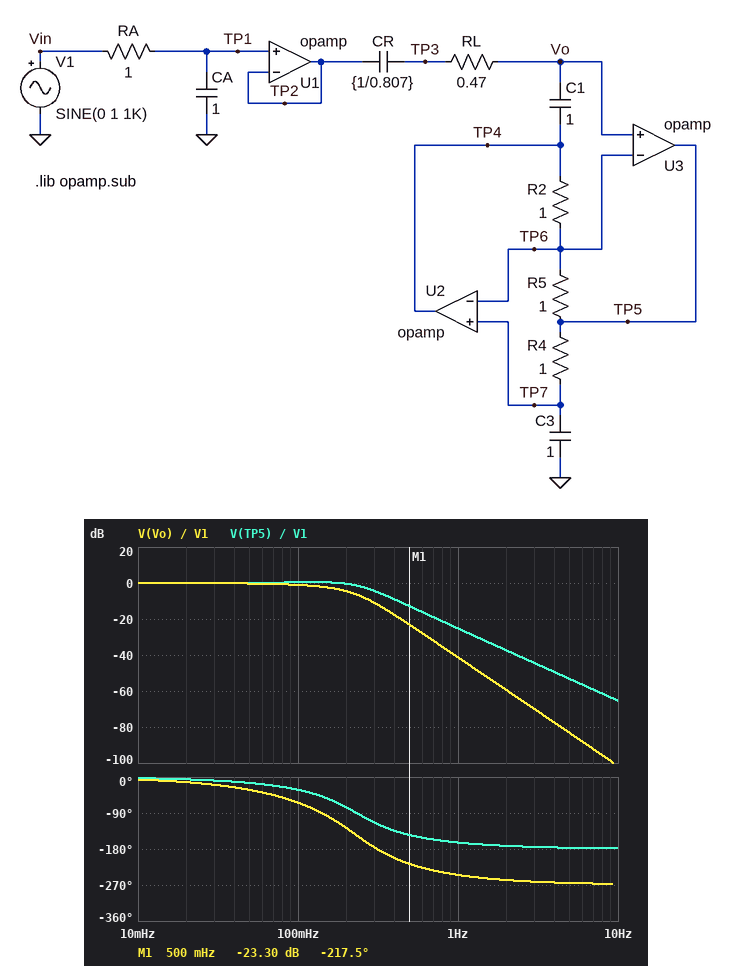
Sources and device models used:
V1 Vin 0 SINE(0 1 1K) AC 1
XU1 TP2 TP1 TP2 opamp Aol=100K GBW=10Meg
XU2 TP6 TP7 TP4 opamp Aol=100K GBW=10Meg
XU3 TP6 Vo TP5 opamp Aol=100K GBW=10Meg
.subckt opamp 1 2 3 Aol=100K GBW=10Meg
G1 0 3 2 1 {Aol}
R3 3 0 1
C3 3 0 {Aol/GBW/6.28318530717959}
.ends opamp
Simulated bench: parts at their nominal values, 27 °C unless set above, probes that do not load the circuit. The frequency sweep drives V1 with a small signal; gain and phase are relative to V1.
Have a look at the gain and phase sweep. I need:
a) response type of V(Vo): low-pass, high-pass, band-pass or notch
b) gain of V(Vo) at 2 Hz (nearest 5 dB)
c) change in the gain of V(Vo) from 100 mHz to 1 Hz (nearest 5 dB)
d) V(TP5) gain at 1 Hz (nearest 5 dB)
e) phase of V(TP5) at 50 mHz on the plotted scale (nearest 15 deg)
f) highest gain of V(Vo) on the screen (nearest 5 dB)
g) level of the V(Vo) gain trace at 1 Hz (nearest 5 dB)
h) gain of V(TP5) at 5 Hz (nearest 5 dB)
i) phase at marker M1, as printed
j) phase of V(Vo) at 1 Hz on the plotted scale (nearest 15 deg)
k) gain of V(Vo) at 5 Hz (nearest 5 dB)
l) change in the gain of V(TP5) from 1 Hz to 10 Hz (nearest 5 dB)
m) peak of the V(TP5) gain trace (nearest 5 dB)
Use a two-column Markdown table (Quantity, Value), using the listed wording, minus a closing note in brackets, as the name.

| Quantity | Value |
|---|---|
| response type of V(Vo): low-pass, high-pass, band-pass or notch | low-pass |
| gain of V(Vo) at 2 Hz | -60 dB |
| change in the gain of V(Vo) from 100 mHz to 1 Hz | -40 dB |
| V(TP5) gain at 1 Hz | -25 dB |
| phase of V(TP5) at 50 mHz on the plotted scale | -15 deg |
| highest gain of V(Vo) on the screen | 0 dB |
| level of the V(Vo) gain trace at 1 Hz | -40 dB |
| gain of V(TP5) at 5 Hz | -55 dB |
| phase at marker M1, as printed | -217.5 deg |
| phase of V(Vo) at 1 Hz on the plotted scale | -240 deg |
| gain of V(Vo) at 5 Hz | -85 dB |
| change in the gain of V(TP5) from 1 Hz to 10 Hz | -40 dB |
| peak of the V(TP5) gain trace | 0 dB |
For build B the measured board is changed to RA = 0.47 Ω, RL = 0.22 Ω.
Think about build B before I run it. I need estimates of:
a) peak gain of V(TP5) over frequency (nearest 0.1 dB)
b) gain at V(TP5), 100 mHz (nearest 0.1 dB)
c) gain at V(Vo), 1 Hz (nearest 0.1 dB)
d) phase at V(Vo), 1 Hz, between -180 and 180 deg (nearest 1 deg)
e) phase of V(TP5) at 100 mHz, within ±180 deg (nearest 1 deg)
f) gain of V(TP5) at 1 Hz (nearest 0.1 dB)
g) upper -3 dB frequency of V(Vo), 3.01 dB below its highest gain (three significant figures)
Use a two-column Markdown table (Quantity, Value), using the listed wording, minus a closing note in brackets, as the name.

| Quantity | Value |
|---|---|
| peak gain of V(TP5) over frequency | 1.2 dB |
| gain at V(TP5), 100 mHz | 0.7 dB |
| gain at V(Vo), 1 Hz | -29.2 dB |
| phase at V(Vo), 1 Hz, between -180 and 180 deg | 142 deg |
| phase of V(TP5) at 100 mHz, within ±180 deg | -13 deg |
| gain of V(TP5) at 1 Hz | -13.1 dB |
| upper -3 dB frequency of V(Vo), 3.01 dB below its highest gain | 203 mHz |
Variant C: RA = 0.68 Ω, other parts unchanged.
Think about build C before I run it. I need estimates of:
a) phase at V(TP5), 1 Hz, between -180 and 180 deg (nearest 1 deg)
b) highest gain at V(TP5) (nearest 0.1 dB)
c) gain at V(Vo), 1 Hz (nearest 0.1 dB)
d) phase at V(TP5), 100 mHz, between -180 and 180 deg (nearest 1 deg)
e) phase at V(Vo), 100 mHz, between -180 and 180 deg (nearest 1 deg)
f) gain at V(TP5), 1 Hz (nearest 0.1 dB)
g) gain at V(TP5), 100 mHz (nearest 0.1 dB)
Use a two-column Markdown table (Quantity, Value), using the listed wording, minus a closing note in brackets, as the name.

| Quantity | Value |
|---|---|
| phase at V(TP5), 1 Hz, between -180 and 180 deg | -160 deg |
| highest gain at V(TP5) | 1.7 dB |
| gain at V(Vo), 1 Hz | -38.1 dB |
| phase at V(TP5), 100 mHz, between -180 and 180 deg | -23 deg |
| phase at V(Vo), 100 mHz, between -180 and 180 deg | -55 deg |
| gain at V(TP5), 1 Hz | -22.0 dB |
| gain at V(TP5), 100 mHz | 1.1 dB |
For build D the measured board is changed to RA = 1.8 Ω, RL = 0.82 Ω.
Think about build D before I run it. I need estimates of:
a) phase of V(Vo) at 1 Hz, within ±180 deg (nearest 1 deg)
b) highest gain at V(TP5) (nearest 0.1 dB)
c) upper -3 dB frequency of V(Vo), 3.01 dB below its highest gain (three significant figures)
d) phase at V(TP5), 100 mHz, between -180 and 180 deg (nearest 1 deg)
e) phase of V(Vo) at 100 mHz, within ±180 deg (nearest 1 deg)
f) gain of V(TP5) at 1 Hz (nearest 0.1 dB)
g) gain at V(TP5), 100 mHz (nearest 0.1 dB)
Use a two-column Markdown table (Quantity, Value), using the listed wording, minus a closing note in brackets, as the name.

| Quantity | Value |
|---|---|
| phase of V(Vo) at 1 Hz, within ±180 deg | 104 deg |
| highest gain at V(TP5) | 0 dB |
| upper -3 dB frequency of V(Vo), 3.01 dB below its highest gain | 129 mHz |
| phase at V(TP5), 100 mHz, between -180 and 180 deg | -53 deg |
| phase of V(Vo) at 100 mHz, within ±180 deg | -85 deg |
| gain of V(TP5) at 1 Hz | -35.1 dB |
| gain at V(TP5), 100 mHz | -0.7 dB |
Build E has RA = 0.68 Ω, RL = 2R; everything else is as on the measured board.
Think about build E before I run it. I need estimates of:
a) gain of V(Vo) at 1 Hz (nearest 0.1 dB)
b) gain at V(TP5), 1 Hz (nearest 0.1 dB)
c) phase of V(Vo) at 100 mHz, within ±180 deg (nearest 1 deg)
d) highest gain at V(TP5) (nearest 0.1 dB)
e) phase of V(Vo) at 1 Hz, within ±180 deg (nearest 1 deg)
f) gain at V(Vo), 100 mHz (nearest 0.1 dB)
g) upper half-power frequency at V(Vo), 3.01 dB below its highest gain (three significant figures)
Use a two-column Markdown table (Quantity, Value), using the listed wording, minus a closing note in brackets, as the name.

| Quantity | Value |
|---|---|
| gain of V(Vo) at 1 Hz | -50.7 dB |
| gain at V(TP5), 1 Hz | -34.6 dB |
| phase of V(Vo) at 100 mHz, within ±180 deg | -91 deg |
| highest gain at V(TP5) | 6.0 dB |
| phase of V(Vo) at 1 Hz, within ±180 deg | 107 deg |
| gain at V(Vo), 100 mHz | 4.5 dB |
| upper half-power frequency at V(Vo), 3.01 dB below its highest gain | 130 mHz |
